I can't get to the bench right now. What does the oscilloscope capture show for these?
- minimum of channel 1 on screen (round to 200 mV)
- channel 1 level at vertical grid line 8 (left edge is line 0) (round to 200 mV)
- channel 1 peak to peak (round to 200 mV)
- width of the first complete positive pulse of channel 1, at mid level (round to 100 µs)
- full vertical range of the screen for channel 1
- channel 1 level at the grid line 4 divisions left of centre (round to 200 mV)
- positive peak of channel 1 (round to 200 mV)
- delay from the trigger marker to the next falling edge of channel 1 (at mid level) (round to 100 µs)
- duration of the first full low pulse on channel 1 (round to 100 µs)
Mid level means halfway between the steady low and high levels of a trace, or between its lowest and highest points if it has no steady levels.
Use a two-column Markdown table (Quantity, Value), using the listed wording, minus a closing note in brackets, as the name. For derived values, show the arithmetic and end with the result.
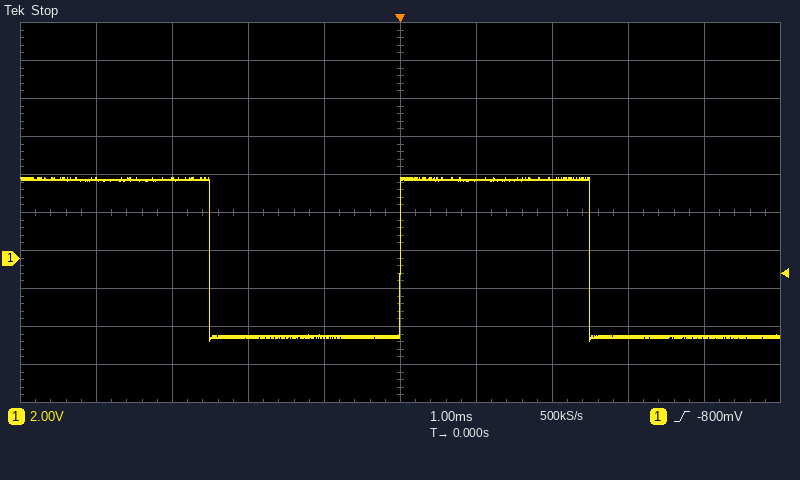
| Quantity | Value |
|---|---|
| minimum of channel 1 on screen | -4.4 V |
| channel 1 level at vertical grid line 8 (left edge is line 0) | -4.2 V |
| channel 1 peak to peak | 4.2 V − (-4.4 V) = 8.6 V |
| width of the first complete positive pulse of channel 1, at mid level | 2.5 ms |
| full vertical range of the screen for channel 1 | 20 V |
| channel 1 level at the grid line 4 divisions left of centre | 4.2 V |
| positive peak of channel 1 | 4.2 V |
| delay from the trigger marker to the next falling edge of channel 1 (at mid level) | 2.5 ms |
| duration of the first full low pulse on channel 1 | 2.5 ms |
